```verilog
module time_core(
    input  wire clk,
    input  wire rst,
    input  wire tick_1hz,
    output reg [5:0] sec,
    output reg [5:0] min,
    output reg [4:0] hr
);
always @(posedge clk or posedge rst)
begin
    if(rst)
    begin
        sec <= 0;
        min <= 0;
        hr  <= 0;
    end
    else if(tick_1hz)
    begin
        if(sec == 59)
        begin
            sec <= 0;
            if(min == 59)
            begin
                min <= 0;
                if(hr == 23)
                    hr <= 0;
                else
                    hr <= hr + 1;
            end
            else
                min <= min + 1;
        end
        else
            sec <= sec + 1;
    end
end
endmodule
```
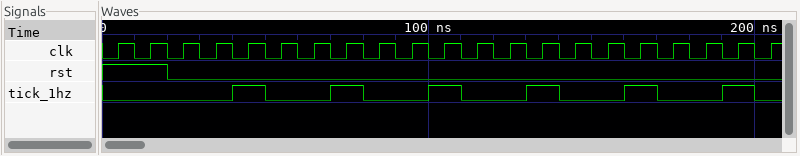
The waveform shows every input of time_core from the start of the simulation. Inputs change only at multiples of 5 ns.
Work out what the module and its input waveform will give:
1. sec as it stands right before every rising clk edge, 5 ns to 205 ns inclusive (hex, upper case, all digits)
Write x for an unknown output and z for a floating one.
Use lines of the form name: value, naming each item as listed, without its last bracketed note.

sec as it stands right before every rising clk edge, 5 ns to 205 ns inclusive: 00, 00, 00, 00, 00, 01, 01, 01, 02, 02, 02, 03, 03, 03, 04, 04, 04, 05, 05, 05, 06
